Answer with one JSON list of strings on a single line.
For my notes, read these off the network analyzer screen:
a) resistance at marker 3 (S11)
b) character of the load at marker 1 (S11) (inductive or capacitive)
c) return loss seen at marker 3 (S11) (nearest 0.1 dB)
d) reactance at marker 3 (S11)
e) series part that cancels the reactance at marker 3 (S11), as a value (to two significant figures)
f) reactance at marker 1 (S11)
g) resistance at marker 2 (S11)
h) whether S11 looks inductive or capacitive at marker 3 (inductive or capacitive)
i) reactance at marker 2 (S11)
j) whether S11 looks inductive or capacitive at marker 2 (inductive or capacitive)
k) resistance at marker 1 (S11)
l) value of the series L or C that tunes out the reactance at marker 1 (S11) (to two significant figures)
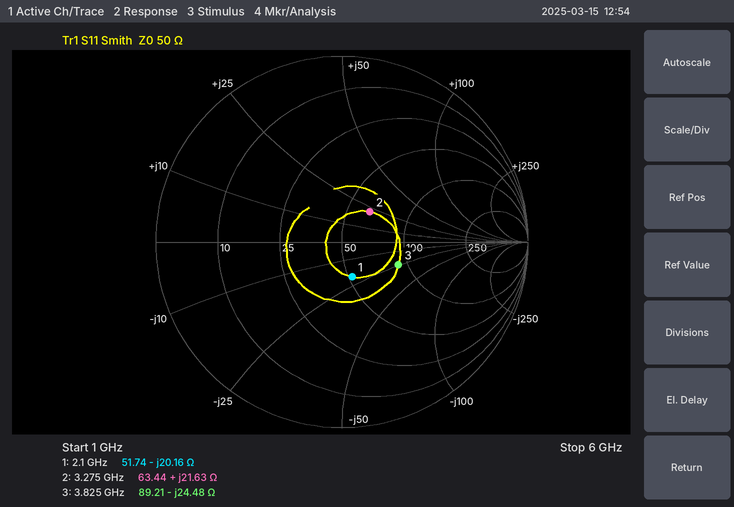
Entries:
["89.21 Ω", "capacitive", "9.7 dB", "-24.48 Ω", "1.0 nH", "-20.16 Ω", "63.44 Ω", "capacitive", "+21.63 Ω", "inductive", "51.74 Ω", "1.5 nH"]
